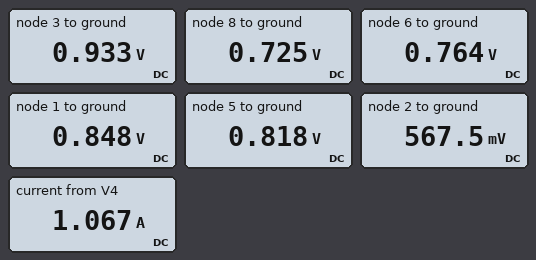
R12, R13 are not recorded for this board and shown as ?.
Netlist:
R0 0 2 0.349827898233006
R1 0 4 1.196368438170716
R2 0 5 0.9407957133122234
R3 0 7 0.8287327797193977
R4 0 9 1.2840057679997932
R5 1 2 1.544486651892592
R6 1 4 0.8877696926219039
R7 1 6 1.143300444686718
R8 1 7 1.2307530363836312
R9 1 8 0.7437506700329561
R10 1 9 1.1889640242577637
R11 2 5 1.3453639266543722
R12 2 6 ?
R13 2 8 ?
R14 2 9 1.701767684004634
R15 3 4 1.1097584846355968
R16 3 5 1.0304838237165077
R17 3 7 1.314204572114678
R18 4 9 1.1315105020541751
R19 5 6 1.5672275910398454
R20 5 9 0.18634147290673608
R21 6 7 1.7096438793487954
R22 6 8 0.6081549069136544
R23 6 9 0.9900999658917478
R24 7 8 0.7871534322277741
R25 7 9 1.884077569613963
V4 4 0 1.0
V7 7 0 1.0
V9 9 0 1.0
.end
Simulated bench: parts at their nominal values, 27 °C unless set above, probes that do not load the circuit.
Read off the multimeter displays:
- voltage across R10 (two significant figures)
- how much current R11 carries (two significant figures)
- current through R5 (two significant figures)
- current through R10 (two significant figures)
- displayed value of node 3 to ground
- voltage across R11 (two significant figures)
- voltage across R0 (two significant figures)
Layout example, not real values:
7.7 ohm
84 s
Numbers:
150 mV
190 mA
180 mA
130 mA
0.933 V
250 mV
570 mV
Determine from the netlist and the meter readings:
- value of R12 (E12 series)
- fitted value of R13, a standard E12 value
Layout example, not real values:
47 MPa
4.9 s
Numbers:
0.47 Ω
0.27 Ω
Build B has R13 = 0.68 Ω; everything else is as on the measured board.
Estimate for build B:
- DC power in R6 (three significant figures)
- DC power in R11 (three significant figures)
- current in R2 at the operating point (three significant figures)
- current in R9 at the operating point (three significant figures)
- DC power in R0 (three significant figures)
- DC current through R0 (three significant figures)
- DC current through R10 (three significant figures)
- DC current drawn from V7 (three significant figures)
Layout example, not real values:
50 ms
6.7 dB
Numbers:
22.2 mW
57.2 mW
867 mA
104 mA
828 mW
1.54 A
118 mA
1.78 A
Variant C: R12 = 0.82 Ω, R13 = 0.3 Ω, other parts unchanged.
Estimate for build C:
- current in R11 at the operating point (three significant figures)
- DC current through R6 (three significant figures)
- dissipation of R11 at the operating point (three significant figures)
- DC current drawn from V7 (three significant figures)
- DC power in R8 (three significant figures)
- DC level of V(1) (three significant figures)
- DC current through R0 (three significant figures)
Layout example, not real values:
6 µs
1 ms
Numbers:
201 mA
167 mA
54.1 mW
1.84 A
17.8 mW
852 mV
1.57 A
